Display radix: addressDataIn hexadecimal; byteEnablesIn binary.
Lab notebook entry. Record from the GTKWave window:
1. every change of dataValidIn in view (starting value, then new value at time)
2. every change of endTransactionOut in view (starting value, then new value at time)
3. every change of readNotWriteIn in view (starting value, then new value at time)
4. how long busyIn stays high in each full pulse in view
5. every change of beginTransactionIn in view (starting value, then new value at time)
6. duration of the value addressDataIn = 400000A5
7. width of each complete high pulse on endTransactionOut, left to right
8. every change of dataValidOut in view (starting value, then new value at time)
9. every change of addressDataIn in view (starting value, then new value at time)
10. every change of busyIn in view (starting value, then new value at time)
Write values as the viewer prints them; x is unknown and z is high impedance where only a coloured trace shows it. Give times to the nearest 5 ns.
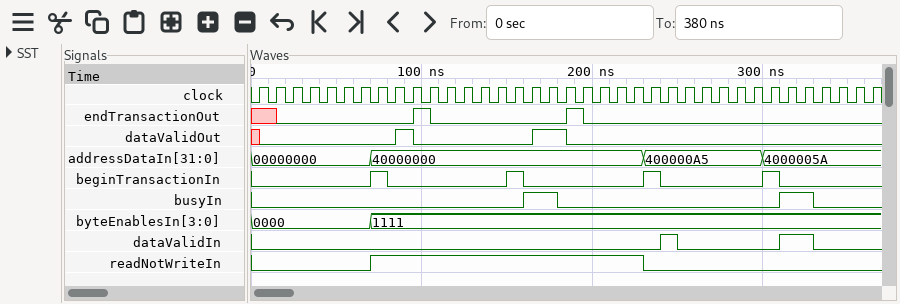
0, 1 at 240 ns, 0 at 250 ns, 1 at 310 ns, 0 at 330 ns
x, 0 at 15 ns, 1 at 95 ns, 0 at 105 ns, 1 at 185 ns, 0 at 195 ns
0, 1 at 70 ns, 0 at 230 ns
20 ns, 20 ns
0, 1 at 70 ns, 0 at 80 ns, 1 at 150 ns, 0 at 160 ns, 1 at 230 ns, 0 at 240 ns, 1 at 300 ns, 0 at 310 ns
70 ns
10 ns, 10 ns
x, 0 at 5 ns, 1 at 85 ns, 0 at 95 ns, 1 at 165 ns, 0 at 185 ns
00000000, 40000000 at 70 ns, 400000A5 at 230 ns, 4000005A at 300 ns
0, 1 at 160 ns, 0 at 180 ns, 1 at 310 ns, 0 at 330 ns
